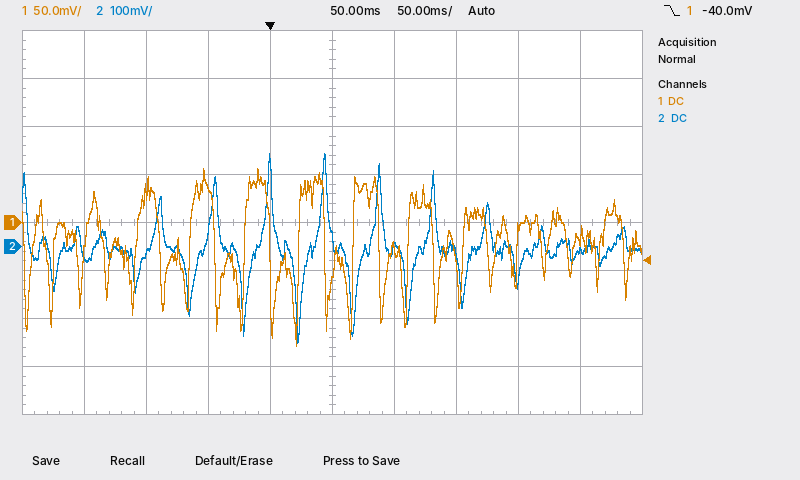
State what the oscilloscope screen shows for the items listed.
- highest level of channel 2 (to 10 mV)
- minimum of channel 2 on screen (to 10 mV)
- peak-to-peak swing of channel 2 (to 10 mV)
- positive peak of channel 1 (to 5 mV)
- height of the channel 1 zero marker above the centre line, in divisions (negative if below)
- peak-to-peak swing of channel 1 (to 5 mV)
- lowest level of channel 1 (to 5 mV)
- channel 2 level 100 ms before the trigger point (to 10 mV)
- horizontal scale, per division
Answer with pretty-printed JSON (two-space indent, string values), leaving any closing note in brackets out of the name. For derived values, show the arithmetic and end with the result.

{
  "highest level of channel 2": "190 mV",
  "minimum of channel 2 on screen": "-200 mV",
  "peak-to-peak swing of channel 2": "190 mV − (-200 mV) = 390 mV",
  "positive peak of channel 1": "55 mV",
  "height of the channel 1 zero marker above the centre line, in divisions": "0.0 div",
  "peak-to-peak swing of channel 1": "55 mV − (-130 mV) = 185 mV",
  "lowest level of channel 1": "-130 mV",
  "channel 2 level 100 ms before the trigger point": "-10 mV",
  "horizontal scale, per division": "50 ms"
}
